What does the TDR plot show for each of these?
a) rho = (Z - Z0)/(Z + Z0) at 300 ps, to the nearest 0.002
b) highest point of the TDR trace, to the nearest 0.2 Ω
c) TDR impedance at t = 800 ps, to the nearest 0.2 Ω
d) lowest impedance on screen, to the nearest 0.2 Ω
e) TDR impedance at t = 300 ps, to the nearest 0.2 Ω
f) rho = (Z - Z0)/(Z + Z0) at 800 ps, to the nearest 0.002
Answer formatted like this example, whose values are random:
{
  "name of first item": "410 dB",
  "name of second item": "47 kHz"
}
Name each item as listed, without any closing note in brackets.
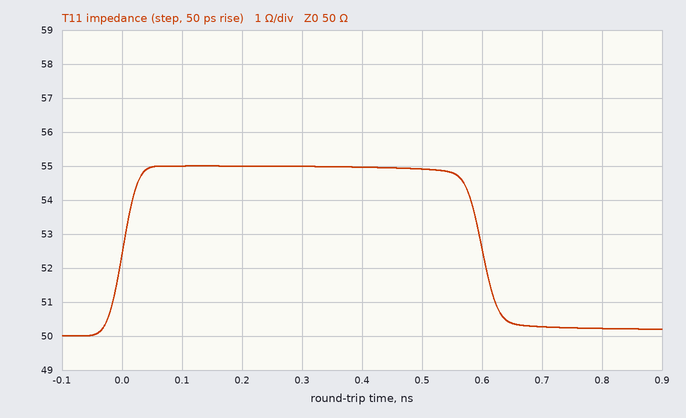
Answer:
{
  "rho = (Z - Z0)/(Z + Z0) at 300 ps, to the nearest 0.002": "+0.048",
  "highest point of the TDR trace, to the nearest 0.2 Ω": "55.0 Ω",
  "TDR impedance at t = 800 ps, to the nearest 0.2 Ω": "50.2 Ω",
  "lowest impedance on screen, to the nearest 0.2 Ω": "50.0 Ω",
  "TDR impedance at t = 300 ps, to the nearest 0.2 Ω": "55.0 Ω",
  "rho = (Z - Z0)/(Z + Z0) at 800 ps, to the nearest 0.002": "+0.002"
}
